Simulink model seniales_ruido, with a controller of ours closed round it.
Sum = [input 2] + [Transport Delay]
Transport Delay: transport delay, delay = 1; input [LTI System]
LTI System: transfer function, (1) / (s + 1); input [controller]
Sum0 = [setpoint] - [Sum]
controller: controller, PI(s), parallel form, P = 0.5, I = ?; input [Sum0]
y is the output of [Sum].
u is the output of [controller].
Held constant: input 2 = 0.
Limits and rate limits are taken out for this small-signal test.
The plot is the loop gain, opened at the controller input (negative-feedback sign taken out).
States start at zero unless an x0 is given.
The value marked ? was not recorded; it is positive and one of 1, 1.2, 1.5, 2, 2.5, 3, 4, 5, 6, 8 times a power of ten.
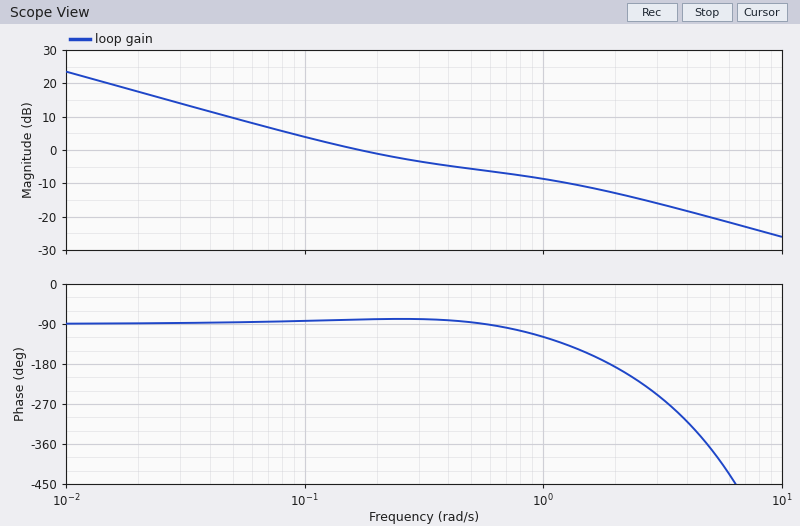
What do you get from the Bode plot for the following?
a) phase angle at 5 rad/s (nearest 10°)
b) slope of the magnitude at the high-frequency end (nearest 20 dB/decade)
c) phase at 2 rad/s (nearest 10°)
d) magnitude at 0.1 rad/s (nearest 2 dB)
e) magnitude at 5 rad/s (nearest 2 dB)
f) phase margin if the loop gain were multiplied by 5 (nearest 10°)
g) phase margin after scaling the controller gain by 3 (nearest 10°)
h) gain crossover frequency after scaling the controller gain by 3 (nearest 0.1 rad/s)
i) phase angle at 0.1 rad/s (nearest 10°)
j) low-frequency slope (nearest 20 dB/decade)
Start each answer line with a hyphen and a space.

- -370°
- -20 dB/decade
- -190°
- 4 dB
- -20 dB
- -30°
- 50°
- 1.2 rad/s
- -80°
- -20 dB/decade
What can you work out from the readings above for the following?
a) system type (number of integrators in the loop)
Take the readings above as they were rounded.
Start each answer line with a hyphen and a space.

- 1
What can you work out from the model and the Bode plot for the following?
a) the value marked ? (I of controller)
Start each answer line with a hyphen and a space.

- 0.15
